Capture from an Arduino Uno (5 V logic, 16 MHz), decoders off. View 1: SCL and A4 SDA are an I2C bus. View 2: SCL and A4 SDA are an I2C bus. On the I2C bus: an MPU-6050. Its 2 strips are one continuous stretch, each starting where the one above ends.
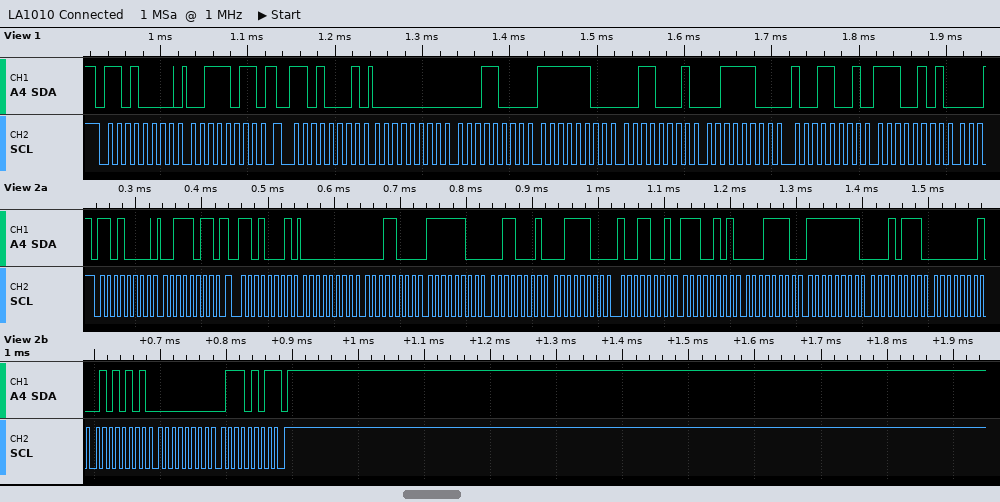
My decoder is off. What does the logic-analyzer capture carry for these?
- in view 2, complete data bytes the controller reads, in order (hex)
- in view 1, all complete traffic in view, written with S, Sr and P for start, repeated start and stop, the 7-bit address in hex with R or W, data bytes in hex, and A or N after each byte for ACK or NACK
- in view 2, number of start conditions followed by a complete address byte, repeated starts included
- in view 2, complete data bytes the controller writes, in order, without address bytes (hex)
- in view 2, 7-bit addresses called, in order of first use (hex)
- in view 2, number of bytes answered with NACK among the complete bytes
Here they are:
00 18 FC 31 3C 99 E5 1E FF 17 01 55 00 75
S 68W A 3B A Sr 68R A 00 A 18 A FC A 31 A 3C A 99 A E5 A
2
3B
0x68
1
